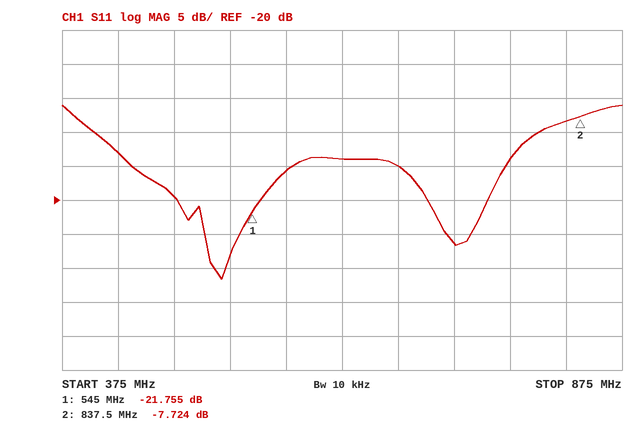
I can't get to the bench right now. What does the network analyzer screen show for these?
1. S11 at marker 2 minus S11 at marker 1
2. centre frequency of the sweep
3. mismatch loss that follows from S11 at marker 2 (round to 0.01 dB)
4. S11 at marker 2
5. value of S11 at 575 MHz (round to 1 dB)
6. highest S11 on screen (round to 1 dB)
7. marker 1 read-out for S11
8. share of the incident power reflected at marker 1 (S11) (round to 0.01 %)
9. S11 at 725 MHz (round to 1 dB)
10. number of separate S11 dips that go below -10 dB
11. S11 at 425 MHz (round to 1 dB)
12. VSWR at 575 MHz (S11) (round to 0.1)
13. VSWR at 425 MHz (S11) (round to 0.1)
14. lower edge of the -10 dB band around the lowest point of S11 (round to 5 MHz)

14.031 dB
625 MHz
0.80 dB
-7.724 dB
-16 dB
-6 dB
-21.755 dB
0.67 %
-26 dB
2
-13 dB
1.4
1.6
405 MHz
